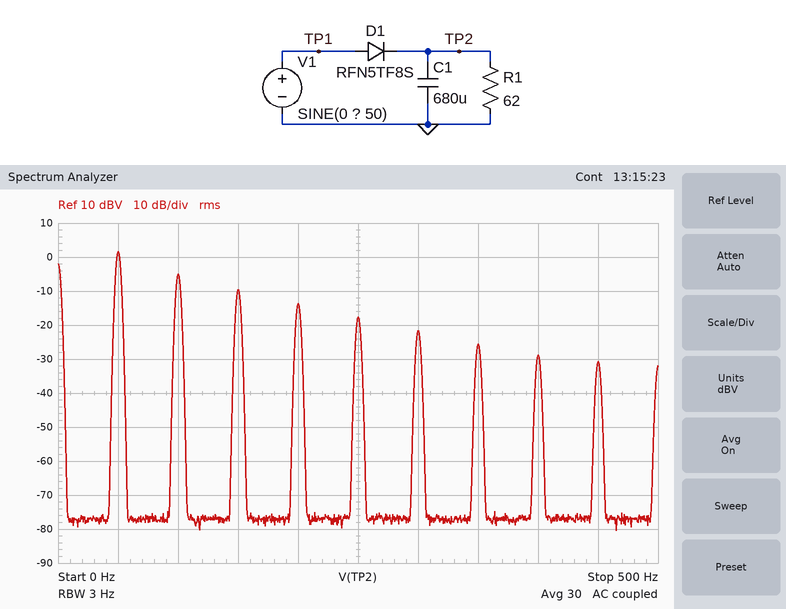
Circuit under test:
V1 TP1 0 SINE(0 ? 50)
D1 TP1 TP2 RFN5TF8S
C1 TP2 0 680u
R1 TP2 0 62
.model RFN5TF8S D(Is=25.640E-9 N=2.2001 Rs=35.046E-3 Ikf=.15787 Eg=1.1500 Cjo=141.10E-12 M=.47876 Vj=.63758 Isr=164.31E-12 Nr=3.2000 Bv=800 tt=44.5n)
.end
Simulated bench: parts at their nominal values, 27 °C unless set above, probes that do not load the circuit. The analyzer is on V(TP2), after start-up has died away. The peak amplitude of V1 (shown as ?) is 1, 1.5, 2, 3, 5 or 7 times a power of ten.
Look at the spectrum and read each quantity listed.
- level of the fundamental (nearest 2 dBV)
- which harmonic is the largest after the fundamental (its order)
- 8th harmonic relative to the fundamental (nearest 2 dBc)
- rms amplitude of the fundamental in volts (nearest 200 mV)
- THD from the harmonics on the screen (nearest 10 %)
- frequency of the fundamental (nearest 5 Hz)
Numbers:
2 dBV
2
-30 dBc
1.2 V
60 %
50 Hz
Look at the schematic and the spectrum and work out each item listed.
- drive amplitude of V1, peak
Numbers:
15 V
